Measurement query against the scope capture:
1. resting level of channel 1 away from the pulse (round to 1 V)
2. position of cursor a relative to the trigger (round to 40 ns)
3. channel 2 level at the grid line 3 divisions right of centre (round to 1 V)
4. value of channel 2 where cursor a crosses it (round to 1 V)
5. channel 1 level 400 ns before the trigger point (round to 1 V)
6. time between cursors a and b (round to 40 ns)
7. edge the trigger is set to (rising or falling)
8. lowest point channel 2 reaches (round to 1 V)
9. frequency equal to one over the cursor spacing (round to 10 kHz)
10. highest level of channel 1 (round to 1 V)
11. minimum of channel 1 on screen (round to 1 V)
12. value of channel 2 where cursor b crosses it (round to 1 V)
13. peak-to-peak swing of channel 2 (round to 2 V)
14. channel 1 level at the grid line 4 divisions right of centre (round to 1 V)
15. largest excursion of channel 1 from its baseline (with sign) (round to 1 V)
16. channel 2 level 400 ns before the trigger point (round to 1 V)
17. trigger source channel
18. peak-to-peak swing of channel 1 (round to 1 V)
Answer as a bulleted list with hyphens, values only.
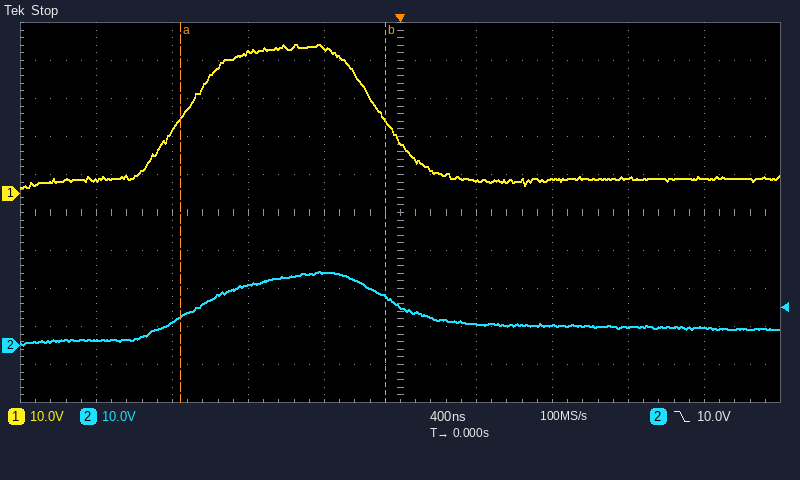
- 4 V
- -1.16 µs
- 5 V
- 8 V
- 38 V
- 1.08 µs
- falling
- 0 V
- 930 kHz
- 39 V
- 1 V
- 13 V
- 20 V
- 4 V
- +35 V
- 19 V
- channel 2
- 38 V
